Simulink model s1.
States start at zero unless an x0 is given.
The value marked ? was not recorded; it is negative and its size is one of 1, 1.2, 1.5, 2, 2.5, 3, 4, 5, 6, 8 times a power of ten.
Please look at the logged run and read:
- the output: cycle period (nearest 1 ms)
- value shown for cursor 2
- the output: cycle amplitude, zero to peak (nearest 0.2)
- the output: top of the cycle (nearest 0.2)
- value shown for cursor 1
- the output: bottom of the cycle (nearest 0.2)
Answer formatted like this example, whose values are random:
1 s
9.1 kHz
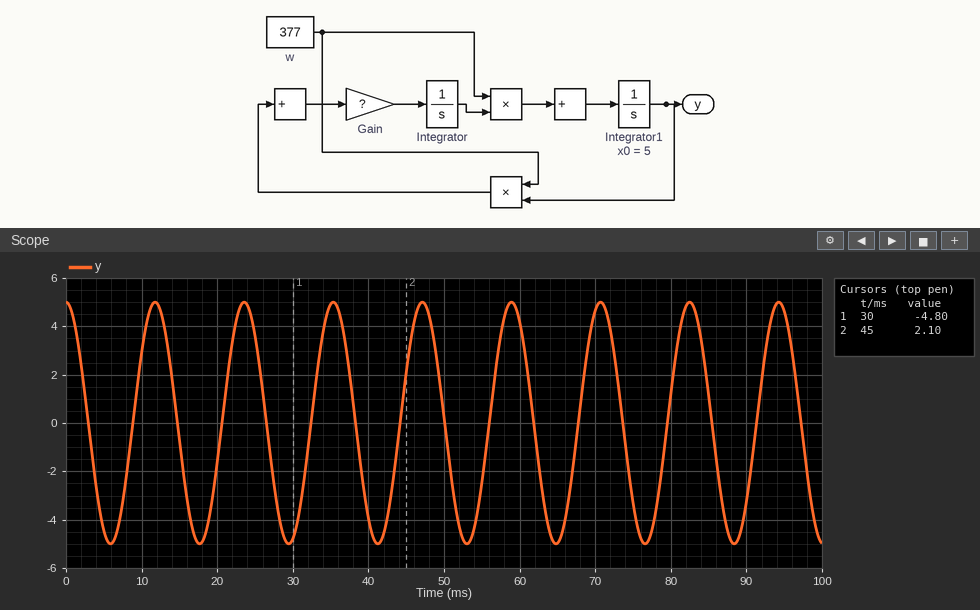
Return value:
12 ms
2.10
5.0
5.0
-4.80
-5.0
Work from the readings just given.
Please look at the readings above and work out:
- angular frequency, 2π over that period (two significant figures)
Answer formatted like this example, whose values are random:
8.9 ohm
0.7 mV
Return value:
0.52 rad/ms
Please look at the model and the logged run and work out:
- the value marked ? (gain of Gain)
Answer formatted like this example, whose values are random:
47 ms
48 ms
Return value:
-2
